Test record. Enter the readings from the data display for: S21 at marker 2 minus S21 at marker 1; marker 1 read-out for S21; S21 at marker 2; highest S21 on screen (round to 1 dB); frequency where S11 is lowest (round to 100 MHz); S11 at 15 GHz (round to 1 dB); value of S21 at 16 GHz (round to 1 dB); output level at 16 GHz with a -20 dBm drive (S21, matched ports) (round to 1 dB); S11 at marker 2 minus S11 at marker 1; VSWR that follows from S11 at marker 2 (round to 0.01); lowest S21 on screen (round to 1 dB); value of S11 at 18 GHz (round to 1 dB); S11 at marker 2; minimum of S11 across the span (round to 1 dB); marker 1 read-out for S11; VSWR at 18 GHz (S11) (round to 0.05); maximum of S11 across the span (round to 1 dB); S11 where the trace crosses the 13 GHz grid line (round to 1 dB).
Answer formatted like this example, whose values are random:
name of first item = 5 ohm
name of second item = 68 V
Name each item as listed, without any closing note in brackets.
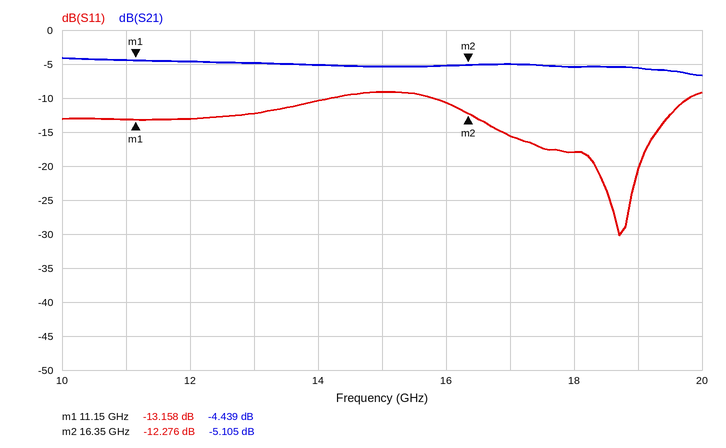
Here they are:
S21 at marker 2 minus S21 at marker 1 = -0.666 dB
marker 1 read-out for S21 = -4.439 dB
S21 at marker 2 = -5.105 dB
highest S21 on screen = -4 dB
frequency where S11 is lowest = 18.7 GHz
S11 at 15 GHz = -9 dB
value of S21 at 16 GHz = -5 dB
output level at 16 GHz with a -20 dBm drive (S21, matched ports) = -25 dBm
S11 at marker 2 minus S11 at marker 1 = 0.882 dB
VSWR that follows from S11 at marker 2 = 1.64
lowest S21 on screen = -7 dB
value of S11 at 18 GHz = -18 dB
S11 at marker 2 = -12.276 dB
minimum of S11 across the span = -30 dB
marker 1 read-out for S11 = -13.158 dB
VSWR at 18 GHz (S11) = 1.30
maximum of S11 across the span = -9 dB
S11 where the trace crosses the 13 GHz grid line = -12 dB
